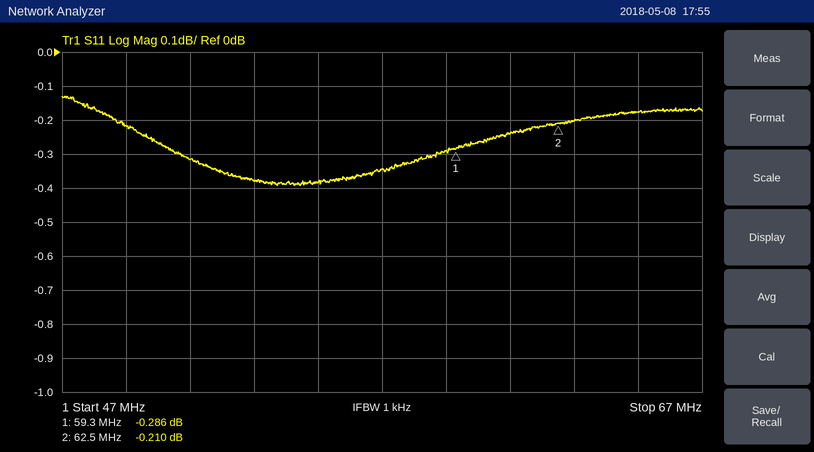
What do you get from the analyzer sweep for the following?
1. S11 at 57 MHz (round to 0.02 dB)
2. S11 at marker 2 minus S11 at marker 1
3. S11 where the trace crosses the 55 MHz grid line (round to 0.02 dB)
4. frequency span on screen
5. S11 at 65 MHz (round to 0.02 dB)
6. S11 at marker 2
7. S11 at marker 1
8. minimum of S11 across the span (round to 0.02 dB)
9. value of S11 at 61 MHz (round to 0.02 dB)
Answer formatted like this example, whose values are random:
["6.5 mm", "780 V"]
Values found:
["-0.34 dB", "0.076 dB", "-0.38 dB", "20 MHz", "-0.18 dB", "-0.210 dB", "-0.286 dB", "-0.40 dB", "-0.24 dB"]
